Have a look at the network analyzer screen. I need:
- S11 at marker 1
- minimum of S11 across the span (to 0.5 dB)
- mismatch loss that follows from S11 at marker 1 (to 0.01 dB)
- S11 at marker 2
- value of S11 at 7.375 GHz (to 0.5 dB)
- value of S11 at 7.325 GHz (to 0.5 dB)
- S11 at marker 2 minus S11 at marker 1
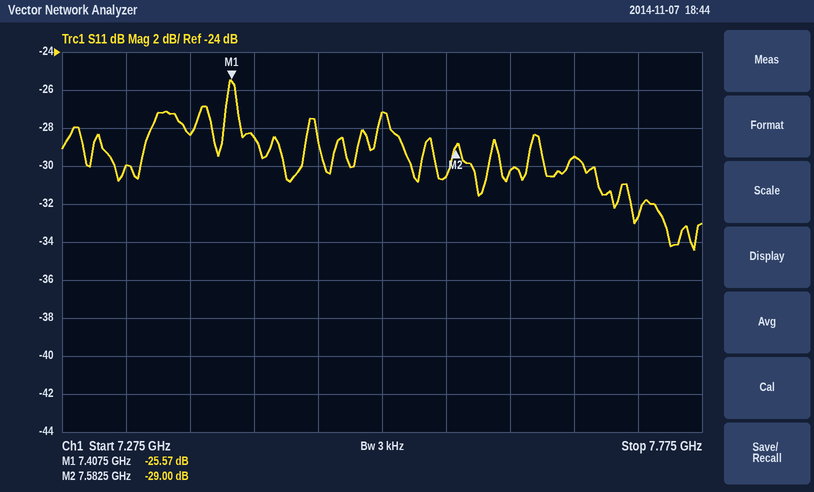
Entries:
-25.57 dB
-34.5 dB
0.01 dB
-29.00 dB
-28.5 dB
-30.0 dB
-3.43 dB
